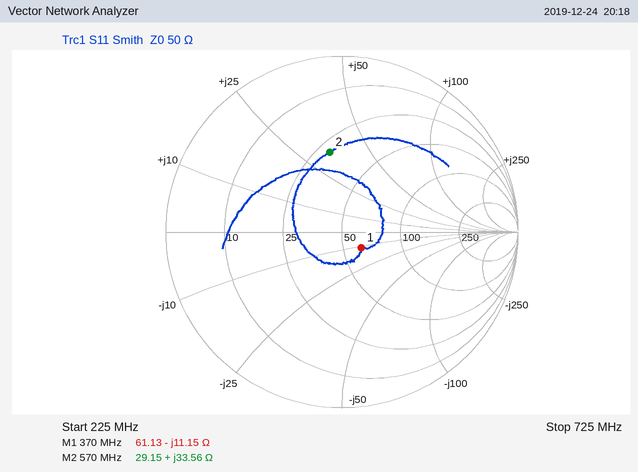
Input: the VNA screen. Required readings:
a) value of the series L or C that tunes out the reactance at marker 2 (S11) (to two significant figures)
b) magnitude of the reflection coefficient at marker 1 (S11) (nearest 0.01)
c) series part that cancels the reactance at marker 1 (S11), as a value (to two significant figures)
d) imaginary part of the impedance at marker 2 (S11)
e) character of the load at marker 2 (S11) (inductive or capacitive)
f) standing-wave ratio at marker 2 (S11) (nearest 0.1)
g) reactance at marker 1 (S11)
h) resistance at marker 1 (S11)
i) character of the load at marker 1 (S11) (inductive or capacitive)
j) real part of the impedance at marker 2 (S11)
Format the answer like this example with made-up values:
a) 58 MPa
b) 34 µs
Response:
a) 8.3 pF
b) 0.14
c) 4.8 nH
d) +33.56 Ω
e) inductive
f) 2.7
g) -11.15 Ω
h) 61.13 Ω
i) capacitive
j) 29.15 Ω
